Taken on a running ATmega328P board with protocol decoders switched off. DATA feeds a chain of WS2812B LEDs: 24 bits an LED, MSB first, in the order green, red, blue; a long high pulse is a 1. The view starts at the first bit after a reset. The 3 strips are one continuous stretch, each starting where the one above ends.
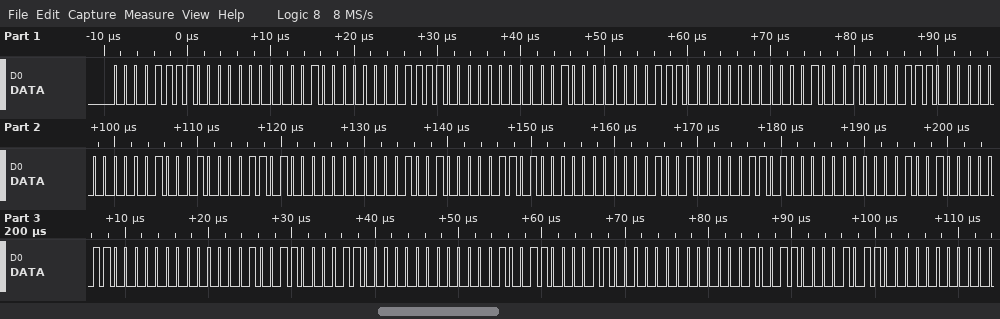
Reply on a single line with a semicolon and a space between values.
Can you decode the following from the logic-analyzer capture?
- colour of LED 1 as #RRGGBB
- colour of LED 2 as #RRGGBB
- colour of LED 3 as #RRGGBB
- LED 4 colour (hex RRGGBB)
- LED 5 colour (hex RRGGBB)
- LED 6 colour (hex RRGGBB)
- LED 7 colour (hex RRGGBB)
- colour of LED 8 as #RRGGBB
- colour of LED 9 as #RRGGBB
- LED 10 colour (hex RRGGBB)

#000F10; #000F10; #000E11; #000E11; #000D12; #000D12; #000D12; #000C13; #000C13; #000C13
